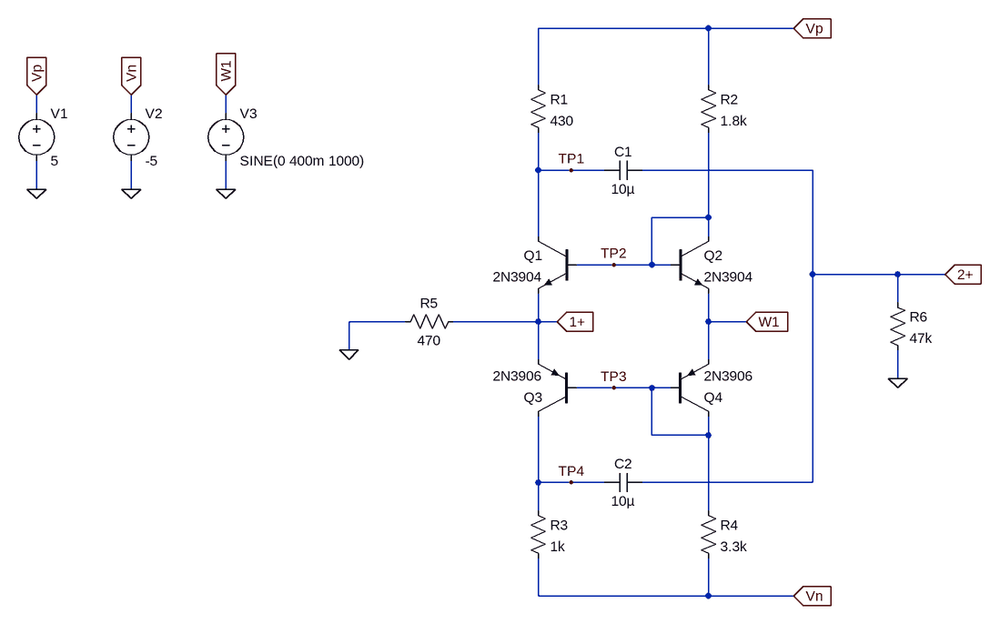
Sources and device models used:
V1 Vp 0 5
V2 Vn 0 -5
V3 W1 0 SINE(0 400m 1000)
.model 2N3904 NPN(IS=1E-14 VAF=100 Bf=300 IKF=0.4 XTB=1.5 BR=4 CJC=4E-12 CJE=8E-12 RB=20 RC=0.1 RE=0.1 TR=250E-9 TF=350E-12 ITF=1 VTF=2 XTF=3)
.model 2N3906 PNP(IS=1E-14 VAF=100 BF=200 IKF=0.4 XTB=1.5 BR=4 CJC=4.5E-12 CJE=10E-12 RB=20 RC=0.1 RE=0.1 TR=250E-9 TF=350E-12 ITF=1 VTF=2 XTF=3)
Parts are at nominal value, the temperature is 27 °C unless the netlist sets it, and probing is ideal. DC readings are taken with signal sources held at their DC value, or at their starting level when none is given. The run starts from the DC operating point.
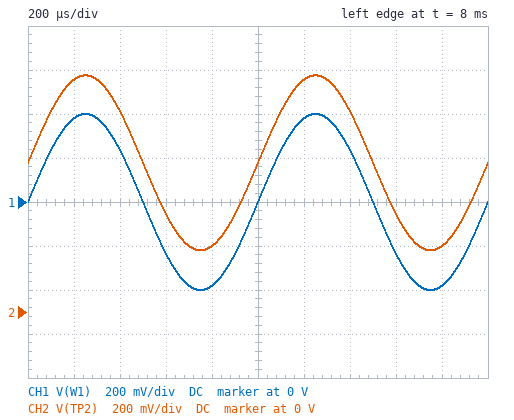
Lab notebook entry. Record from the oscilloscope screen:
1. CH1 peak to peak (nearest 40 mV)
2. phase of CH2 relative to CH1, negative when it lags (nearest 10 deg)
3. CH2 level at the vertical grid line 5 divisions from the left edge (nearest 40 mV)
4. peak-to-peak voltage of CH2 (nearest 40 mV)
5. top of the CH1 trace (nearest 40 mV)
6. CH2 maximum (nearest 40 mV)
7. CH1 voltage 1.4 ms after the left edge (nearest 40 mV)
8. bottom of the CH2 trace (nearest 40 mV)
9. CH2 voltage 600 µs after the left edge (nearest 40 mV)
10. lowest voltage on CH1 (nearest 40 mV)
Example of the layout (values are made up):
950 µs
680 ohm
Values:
800 mV
0 deg
680 mV
800 mV
400 mV
1.08 V
240 mV
280 mV
440 mV
-400 mV
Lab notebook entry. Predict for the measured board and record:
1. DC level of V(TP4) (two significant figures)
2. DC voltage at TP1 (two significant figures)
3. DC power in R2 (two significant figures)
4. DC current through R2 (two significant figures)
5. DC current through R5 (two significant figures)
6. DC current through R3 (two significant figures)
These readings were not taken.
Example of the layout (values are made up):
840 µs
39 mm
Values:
-3.2 V
4.2 V
10 mW
2.4 mA
17 µA
1.8 mA
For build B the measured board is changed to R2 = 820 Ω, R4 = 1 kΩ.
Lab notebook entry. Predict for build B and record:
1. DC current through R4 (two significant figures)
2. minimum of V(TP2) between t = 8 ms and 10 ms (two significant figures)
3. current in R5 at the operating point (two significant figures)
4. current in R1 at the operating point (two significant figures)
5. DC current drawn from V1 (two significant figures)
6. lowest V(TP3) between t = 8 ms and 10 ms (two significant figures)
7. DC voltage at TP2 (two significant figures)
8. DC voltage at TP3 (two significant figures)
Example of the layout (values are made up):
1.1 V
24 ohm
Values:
4.3 mA
300 mV
6.5 µA
4.8 mA
10 mA
-1.1 V
700 mV
-690 mV
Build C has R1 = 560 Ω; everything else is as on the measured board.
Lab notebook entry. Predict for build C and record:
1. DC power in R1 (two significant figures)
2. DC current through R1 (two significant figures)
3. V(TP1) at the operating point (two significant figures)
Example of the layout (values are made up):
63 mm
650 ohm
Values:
1.9 mW
1.8 mA
4.0 V
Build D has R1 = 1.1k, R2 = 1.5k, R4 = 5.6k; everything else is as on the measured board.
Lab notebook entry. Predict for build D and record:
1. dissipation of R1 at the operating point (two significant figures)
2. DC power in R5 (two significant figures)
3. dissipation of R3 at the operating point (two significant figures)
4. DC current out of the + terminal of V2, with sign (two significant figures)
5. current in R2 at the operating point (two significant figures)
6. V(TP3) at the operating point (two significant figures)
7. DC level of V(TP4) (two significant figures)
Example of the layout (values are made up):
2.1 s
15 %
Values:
2.6 mW
610 nW
2.3 mW
-2.3 mA
2.9 mA
-650 mV
-3.5 V
